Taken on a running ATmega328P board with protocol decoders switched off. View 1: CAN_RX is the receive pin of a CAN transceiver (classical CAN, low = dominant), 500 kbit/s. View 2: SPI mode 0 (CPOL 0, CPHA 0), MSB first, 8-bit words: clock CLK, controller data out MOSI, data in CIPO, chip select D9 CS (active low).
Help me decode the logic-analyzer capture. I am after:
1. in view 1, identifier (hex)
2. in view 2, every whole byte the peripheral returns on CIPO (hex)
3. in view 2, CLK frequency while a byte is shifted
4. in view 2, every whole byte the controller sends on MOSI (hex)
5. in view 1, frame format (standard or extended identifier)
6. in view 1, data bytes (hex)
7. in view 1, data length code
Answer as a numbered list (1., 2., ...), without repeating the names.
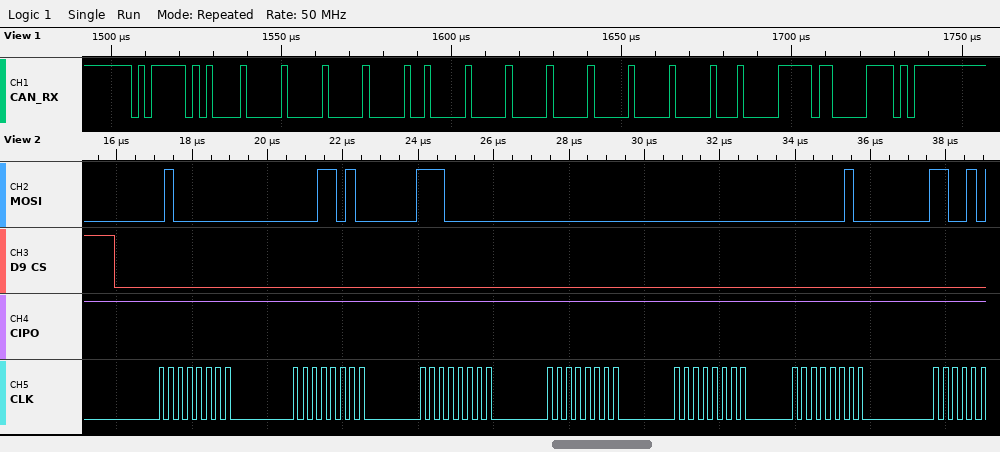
1. 0x5FA
2. 0xFF 0xFF 0xFF 0xFF 0xFF 0xFF
3. 4 MHz
4. 0x40 0x1A 0xE0 0x00 0x00 0x02
5. standard
6. 00 00 10 00 00 00 00 20
7. 8
